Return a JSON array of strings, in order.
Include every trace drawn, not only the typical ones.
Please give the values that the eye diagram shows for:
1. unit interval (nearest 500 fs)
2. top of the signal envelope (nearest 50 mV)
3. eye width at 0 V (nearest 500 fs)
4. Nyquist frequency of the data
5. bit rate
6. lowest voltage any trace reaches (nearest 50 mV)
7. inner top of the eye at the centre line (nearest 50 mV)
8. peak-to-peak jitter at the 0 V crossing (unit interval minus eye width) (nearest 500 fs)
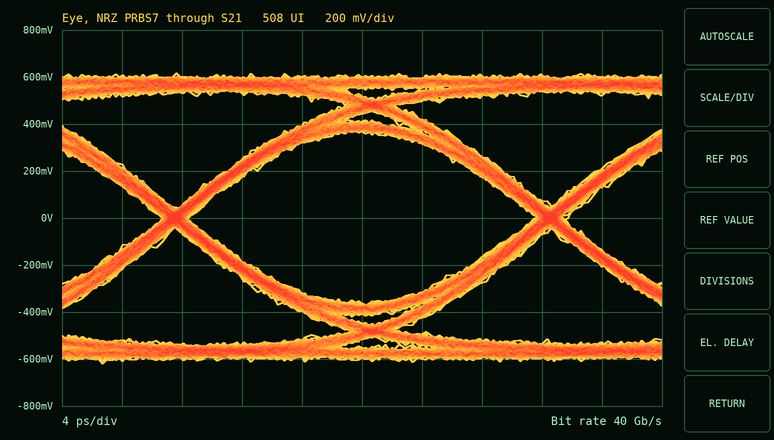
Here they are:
["25.0 ps", "600 mV", "23.0 ps", "20 GHz", "40 Gb/s", "-600 mV", "350 mV", "2.0 ps"]
